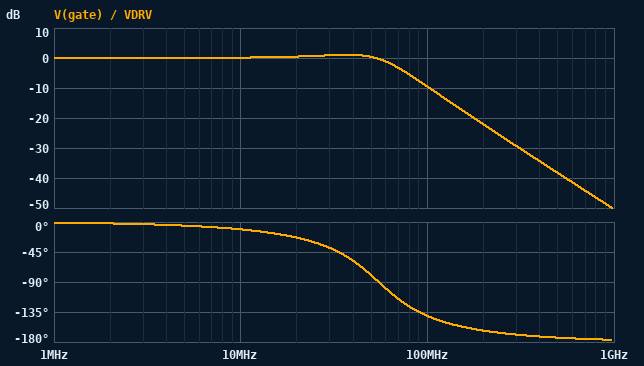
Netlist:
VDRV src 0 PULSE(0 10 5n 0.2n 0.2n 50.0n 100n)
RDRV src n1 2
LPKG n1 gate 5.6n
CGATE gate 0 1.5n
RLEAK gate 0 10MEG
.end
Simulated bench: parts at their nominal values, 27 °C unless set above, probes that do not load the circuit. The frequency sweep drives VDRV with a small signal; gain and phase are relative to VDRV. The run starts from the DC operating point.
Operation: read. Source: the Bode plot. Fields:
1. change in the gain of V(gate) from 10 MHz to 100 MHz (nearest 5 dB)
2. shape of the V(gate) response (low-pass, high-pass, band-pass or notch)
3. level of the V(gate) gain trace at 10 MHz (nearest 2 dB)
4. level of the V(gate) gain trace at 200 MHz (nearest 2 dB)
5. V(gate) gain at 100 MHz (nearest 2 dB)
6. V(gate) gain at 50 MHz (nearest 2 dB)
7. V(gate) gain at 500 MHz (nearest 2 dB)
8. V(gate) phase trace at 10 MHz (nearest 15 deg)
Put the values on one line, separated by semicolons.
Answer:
-10 dB; low-pass; 0 dB; -22 dB; -10 dB; 0 dB; -38 dB; -15 deg
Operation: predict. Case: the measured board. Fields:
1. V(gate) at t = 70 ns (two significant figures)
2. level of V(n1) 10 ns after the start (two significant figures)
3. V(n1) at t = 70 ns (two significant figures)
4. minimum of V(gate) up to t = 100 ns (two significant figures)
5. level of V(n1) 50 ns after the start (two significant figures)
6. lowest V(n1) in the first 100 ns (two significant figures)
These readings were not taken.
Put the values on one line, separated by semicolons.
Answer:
-670 mV; 5.0 V; -820 mV; -1.5 V; 10 V; -830 mV
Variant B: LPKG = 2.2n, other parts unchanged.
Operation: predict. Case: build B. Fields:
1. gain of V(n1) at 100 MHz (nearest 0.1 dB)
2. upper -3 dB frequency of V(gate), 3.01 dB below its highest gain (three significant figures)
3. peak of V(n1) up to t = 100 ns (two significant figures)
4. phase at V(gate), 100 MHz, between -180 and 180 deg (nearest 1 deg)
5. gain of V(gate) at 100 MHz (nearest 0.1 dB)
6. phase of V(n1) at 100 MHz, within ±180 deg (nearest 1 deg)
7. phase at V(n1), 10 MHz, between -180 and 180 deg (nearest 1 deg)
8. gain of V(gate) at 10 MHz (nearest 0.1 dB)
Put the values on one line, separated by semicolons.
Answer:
-16.0 dB; 73.3 MHz; 10 V; -99 deg; -5.6 dB; 81 deg; -11 deg; 0 dB
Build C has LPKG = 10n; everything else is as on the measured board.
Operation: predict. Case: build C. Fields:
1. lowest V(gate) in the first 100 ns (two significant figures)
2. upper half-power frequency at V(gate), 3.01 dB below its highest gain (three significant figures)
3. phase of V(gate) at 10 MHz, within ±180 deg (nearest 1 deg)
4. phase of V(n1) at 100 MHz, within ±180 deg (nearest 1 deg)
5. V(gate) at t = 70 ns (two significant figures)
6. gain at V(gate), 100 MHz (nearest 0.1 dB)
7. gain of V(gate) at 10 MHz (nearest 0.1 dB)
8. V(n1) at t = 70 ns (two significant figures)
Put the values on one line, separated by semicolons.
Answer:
-2.7 V; 48.9 MHz; -11 deg; 21 deg; -2.5 V; -14.4 dB; 0.4 dB; -680 mV
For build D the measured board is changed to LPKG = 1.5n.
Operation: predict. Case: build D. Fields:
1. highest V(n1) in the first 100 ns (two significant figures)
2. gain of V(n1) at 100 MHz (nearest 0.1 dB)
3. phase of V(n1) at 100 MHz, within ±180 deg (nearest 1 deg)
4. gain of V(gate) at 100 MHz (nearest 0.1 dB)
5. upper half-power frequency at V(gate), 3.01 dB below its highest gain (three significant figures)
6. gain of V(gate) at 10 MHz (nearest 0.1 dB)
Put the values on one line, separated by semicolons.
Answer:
10 V; -24.6 dB; -87 deg; -5.5 dB; 68.3 MHz; -0.1 dB
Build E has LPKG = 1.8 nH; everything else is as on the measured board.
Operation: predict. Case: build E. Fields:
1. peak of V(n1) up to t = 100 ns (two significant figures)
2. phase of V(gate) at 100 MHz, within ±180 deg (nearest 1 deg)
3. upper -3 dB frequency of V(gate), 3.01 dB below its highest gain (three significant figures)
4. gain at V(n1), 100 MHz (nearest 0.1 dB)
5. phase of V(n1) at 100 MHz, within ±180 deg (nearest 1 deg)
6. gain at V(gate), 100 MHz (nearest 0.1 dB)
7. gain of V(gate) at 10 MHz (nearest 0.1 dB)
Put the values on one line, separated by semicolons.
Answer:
10 V; -92 deg; 70.9 MHz; -29.1 dB; 88 deg; -5.5 dB; -0.1 dB
